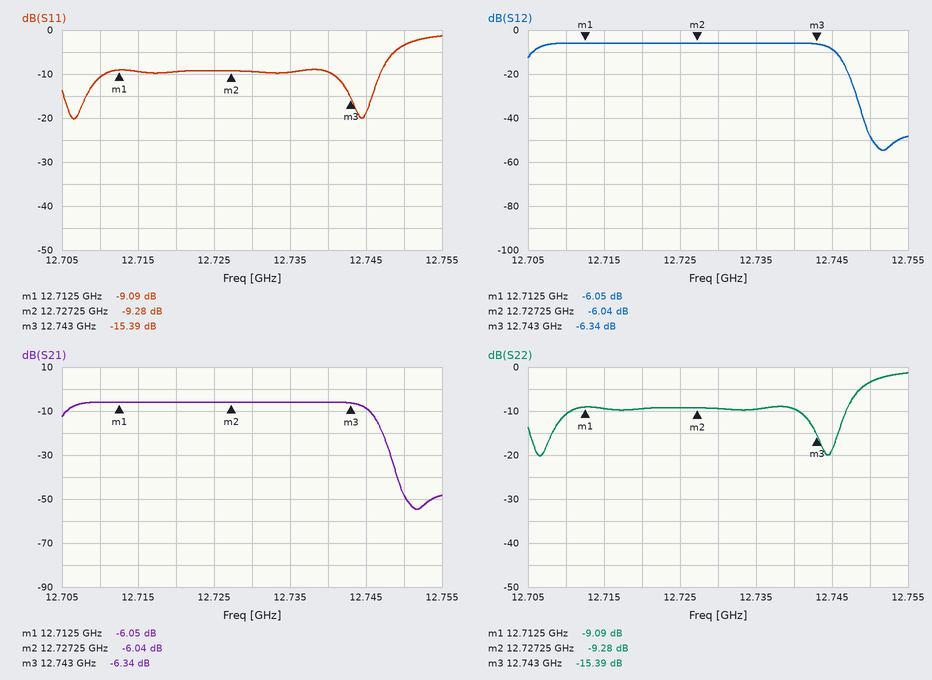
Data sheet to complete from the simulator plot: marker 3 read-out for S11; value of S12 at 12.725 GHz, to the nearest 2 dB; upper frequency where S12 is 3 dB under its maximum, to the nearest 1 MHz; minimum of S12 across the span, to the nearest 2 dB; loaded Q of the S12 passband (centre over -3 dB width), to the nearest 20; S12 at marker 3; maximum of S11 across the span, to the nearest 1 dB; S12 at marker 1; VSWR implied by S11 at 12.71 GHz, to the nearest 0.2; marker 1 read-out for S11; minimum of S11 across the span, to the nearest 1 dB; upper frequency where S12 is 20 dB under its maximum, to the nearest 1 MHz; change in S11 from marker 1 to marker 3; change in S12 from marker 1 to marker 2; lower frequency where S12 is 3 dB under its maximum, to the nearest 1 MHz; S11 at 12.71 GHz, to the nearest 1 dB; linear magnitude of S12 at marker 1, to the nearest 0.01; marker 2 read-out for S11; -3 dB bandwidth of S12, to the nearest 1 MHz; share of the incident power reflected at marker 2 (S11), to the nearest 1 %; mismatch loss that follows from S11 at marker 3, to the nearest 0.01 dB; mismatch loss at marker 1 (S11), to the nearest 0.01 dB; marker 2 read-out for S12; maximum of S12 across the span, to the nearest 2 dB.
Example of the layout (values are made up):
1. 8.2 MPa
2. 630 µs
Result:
1. -15.39 dB
2. -6 dB
3. 12.745 GHz
4. -54 dB
5. 320
6. -6.34 dB
7. -1 dB
8. -6.05 dB
9. 1.8
10. -9.09 dB
11. -20 dB
12. 12.748 GHz
13. -6.30 dB
14. 0.01 dB
15. 12.706 GHz
16. -11 dB
17. 0.50
18. -9.28 dB
19. 39 MHz
20. 12 %
21. 0.13 dB
22. 0.57 dB
23. -6.04 dB
24. -6 dB
